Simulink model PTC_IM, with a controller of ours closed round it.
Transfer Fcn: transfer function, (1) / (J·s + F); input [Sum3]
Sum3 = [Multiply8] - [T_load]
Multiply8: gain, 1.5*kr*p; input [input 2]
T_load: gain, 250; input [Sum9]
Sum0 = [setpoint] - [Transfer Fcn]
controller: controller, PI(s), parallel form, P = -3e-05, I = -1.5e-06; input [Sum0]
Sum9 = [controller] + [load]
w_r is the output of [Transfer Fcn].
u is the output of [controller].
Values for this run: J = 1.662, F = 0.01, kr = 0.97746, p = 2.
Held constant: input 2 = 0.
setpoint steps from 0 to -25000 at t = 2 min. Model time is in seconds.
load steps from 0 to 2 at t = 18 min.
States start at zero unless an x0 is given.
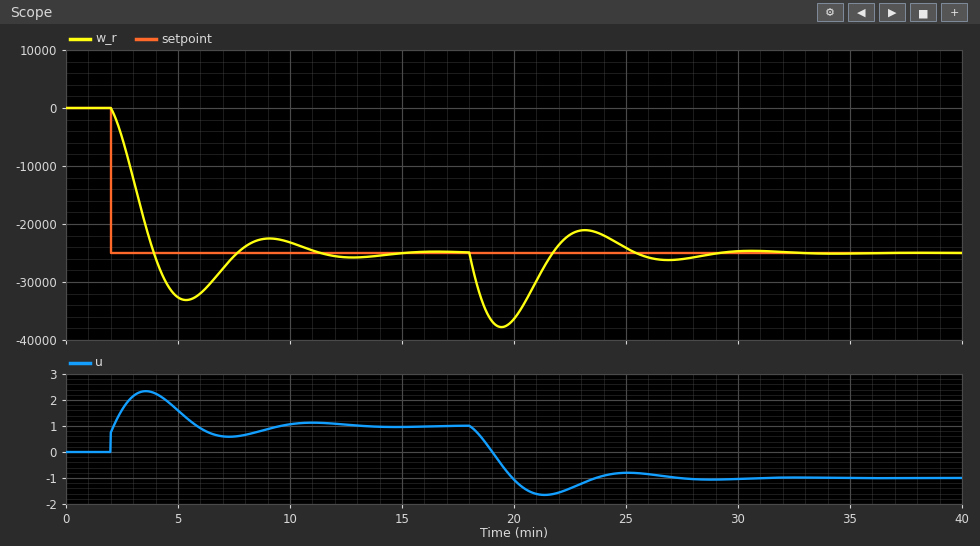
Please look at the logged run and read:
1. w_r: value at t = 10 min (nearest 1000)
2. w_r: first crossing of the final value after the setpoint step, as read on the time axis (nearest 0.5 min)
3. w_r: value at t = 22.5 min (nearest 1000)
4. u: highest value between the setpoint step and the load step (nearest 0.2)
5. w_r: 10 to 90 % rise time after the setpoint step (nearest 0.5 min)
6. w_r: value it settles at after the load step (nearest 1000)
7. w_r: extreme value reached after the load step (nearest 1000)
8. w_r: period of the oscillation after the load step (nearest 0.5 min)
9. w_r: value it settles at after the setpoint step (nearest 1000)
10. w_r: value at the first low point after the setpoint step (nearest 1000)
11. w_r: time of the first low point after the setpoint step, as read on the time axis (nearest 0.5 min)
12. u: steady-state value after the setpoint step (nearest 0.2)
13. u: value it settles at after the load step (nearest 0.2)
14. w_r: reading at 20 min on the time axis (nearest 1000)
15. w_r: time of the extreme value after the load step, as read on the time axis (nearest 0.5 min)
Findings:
-23000
4.0 min
-22000
2.4
1.5 min
-25000
-38000
7.5 min
-25000
-33000
5.5 min
1.0
-1.0
-36000
19.5 min
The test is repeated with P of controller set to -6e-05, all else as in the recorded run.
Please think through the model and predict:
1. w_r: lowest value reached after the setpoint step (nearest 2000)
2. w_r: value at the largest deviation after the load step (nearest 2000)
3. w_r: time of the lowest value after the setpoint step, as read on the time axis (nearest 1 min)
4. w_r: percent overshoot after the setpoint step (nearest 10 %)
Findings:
-30000
-36000
5 min
20 %
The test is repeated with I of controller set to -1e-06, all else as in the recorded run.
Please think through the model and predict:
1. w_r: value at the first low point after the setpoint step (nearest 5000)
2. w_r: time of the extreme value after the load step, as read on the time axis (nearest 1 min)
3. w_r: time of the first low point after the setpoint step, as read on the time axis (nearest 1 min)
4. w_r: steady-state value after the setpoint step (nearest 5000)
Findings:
-30000
20 min
6 min
-25000
